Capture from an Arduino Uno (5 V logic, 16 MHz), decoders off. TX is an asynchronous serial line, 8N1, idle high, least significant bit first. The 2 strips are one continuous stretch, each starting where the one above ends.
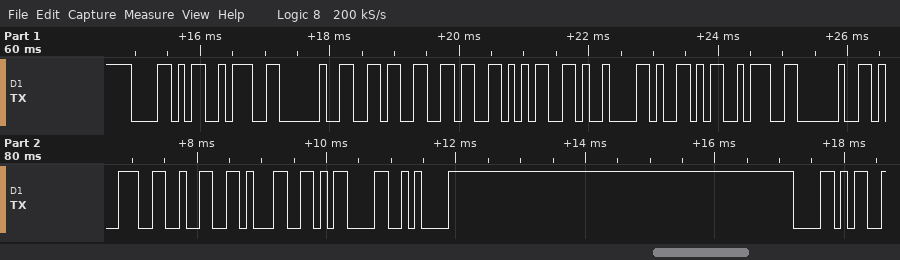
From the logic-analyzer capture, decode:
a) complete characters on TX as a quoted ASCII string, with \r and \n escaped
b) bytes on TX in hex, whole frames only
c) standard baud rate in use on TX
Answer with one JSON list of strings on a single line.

["\"X: 665\\tY: 921\\r\\nX\"", "0x58 0x3A 0x20 0x36 0x36 0x35 0x09 0x59 0x3A 0x20 0x39 0x32 0x31 0x0D 0x0A 0x58", "9600 baud"]
